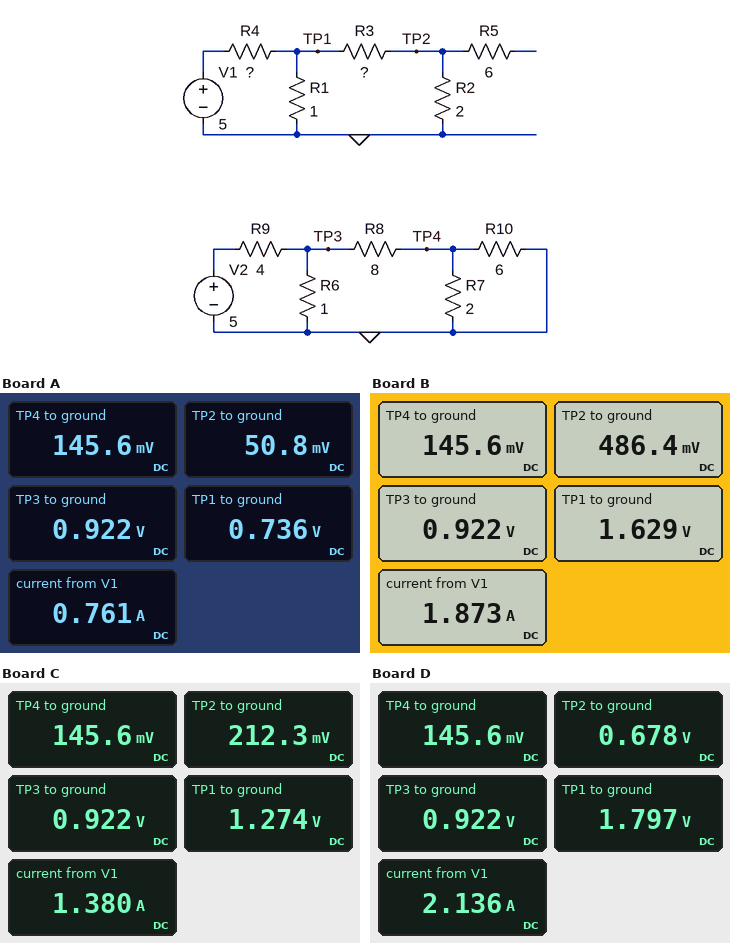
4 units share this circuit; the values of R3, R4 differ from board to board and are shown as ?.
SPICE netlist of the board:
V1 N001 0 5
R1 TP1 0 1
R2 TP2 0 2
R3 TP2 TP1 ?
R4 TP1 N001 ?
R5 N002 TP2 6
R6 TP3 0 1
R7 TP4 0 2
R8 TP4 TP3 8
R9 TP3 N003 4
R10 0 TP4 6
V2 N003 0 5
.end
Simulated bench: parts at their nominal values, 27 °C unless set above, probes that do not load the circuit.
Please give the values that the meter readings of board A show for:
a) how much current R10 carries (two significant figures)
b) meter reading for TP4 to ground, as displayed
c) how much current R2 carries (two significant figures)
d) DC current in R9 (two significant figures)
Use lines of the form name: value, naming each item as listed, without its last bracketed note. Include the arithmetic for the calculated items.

how much current R10 carries: (145.6 mV) / 6 Ω = 24 mA
meter reading for TP4 to ground, as displayed: 145.6 mV
how much current R2 carries: (50.8 mV) / 2 Ω = 25 mA
DC current in R9: (5 V - 922 mV) / 4 Ω = 1.0 A
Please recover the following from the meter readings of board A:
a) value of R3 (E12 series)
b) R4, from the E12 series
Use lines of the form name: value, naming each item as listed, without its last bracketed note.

value of R3: 27 Ω
R4, from the E12 series: 5.6 Ω
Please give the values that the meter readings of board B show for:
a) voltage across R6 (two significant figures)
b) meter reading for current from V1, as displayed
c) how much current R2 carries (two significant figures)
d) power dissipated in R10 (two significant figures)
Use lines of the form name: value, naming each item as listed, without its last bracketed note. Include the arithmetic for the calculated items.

voltage across R6: 922 mV = 920 mV
meter reading for current from V1, as displayed: 1.873 A
how much current R2 carries: (486.4 mV) / 2 Ω = 240 mA
power dissipated in R10: (145.6 mV)^2 / 6 Ω = 3.5 mW
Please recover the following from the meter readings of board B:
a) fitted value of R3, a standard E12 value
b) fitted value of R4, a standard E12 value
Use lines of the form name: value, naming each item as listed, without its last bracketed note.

fitted value of R3, a standard E12 value: 4.7 Ω
fitted value of R4, a standard E12 value: 1.8 Ω
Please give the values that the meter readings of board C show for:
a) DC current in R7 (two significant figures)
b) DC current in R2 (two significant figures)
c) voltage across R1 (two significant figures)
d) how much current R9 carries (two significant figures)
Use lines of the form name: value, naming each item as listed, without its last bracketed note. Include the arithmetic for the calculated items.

DC current in R7: (145.6 mV) / 2 Ω = 73 mA
DC current in R2: (212.3 mV) / 2 Ω = 110 mA
voltage across R1: 1.274 V = 1.3 V
how much current R9 carries: (5 V - 922 mV) / 4 Ω = 1.0 A
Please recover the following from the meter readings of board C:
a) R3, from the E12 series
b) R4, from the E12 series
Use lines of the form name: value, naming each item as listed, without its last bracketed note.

R3, from the E12 series: 10 Ω
R4, from the E12 series: 2.7 Ω
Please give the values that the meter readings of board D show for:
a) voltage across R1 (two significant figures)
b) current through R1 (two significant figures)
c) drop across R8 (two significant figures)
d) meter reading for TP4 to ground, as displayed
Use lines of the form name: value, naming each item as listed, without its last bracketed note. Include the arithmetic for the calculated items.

voltage across R1: 1.797 V = 1.8 V
current through R1: (1.797 V) / 1 Ω = 1.8 A
drop across R8: 922 mV - 145.6 mV = 780 mV
meter reading for TP4 to ground, as displayed: 145.6 mV
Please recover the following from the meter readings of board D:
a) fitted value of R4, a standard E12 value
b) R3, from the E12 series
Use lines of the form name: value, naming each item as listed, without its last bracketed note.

fitted value of R4, a standard E12 value: 1.5 Ω
R3, from the E12 series: 3.3 Ω
